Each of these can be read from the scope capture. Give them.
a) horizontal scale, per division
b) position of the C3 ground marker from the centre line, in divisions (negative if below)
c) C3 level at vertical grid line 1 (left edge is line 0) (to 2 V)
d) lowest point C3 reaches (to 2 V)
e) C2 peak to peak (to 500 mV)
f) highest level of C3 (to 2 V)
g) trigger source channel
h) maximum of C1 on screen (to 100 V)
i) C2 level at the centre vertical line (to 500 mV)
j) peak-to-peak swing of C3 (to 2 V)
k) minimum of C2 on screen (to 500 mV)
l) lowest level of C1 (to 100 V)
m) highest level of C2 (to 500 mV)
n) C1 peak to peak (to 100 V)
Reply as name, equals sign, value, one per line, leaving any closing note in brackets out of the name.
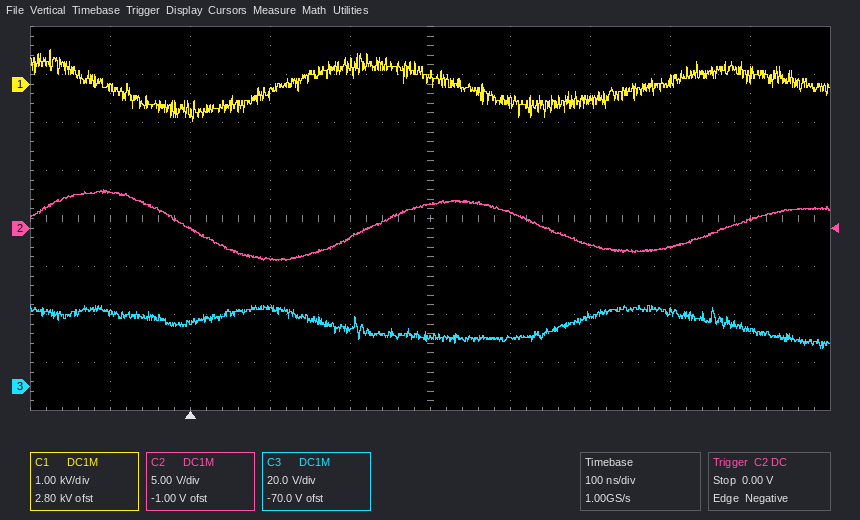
horizontal scale, per division = 100 ns
position of the C3 ground marker from the centre line, in divisions = -3.5 div
C3 level at vertical grid line 1 (left edge is line 0) = 30 V
lowest point C3 reaches = 16 V
C2 peak to peak = 7.5 V
highest level of C3 = 34 V
trigger source channel = C2
maximum of C1 on screen = 700 V
C2 level at the centre vertical line = 2.5 V
peak-to-peak swing of C3 = 18 V
minimum of C2 on screen = -3.5 V
lowest level of C1 = -800 V
highest level of C2 = 4.0 V
C1 peak to peak = 1.5 kV
